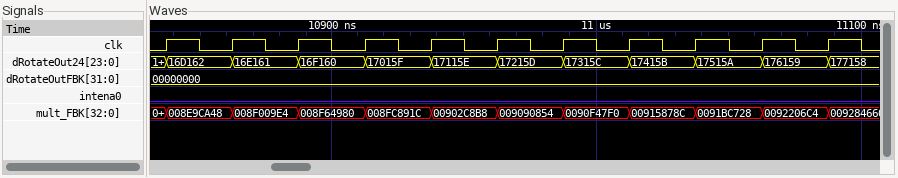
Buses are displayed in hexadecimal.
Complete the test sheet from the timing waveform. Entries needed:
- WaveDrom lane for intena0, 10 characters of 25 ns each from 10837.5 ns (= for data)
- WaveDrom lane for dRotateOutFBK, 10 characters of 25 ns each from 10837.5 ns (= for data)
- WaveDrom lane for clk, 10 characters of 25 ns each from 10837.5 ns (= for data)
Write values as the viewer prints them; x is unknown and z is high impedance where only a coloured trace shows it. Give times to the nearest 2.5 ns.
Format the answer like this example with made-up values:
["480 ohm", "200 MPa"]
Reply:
["{name: 'intena0', wave: '0.........'}", "{name: 'dRotateOutFBK', wave: '=.........', data: '00000000'}", "{name: 'clk', wave: 'p.........'}"]
